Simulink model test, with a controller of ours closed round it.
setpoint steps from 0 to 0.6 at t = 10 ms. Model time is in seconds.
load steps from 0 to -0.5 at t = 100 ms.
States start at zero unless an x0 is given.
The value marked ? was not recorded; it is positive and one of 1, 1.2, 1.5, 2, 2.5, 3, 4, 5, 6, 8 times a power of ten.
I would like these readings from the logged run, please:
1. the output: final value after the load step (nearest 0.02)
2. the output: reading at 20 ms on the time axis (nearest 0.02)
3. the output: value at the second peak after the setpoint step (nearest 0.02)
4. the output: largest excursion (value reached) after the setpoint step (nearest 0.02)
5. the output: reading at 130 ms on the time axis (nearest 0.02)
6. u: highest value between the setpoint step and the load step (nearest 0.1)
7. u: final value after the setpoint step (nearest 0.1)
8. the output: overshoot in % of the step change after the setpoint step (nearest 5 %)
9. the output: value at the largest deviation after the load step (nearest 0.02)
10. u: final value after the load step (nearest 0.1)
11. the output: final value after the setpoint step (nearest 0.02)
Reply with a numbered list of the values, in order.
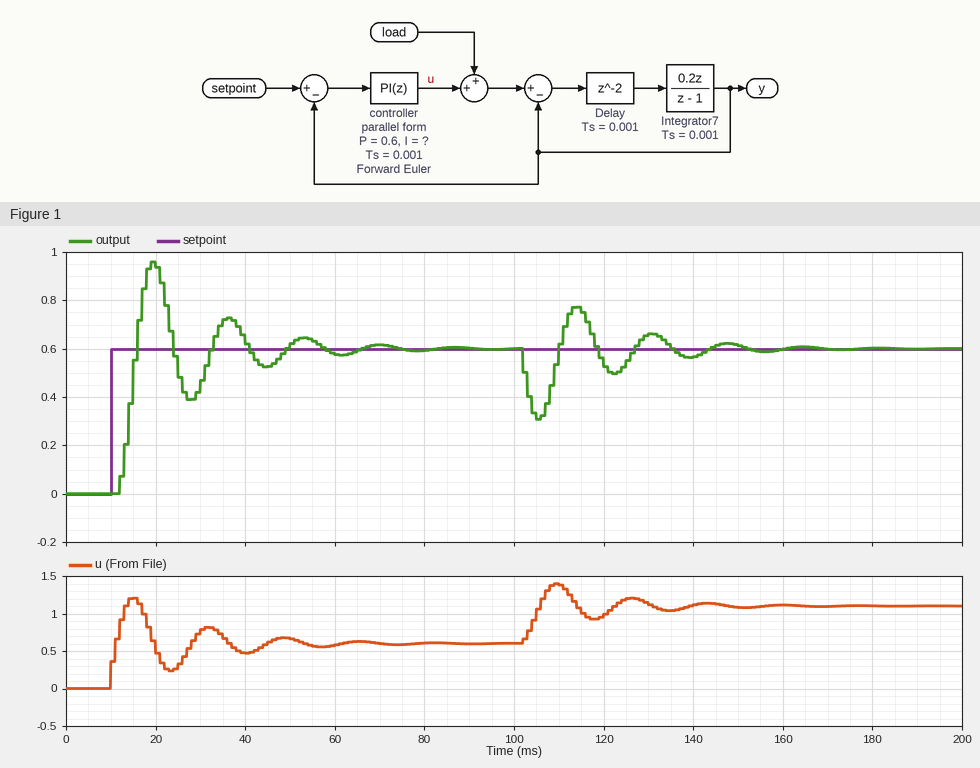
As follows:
1. 0.60
2. 0.94
3. 0.72
4. 0.96
5. 0.66
6. 1.2
7. 0.6
8. 60 %
9. 0.30
10. 1.1
11. 0.60
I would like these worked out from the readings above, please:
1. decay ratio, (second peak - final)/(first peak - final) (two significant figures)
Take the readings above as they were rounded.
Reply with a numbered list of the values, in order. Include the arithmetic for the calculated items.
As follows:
1. (0.72 - 0.6) / (0.96 - 0.6) = 0.33
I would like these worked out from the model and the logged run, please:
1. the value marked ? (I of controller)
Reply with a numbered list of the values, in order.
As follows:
1. 500
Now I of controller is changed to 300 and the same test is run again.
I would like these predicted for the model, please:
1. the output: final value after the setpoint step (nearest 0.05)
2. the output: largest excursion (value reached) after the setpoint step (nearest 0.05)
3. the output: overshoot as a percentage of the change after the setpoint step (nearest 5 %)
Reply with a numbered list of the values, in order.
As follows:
1. 0.60
2. 0.75
3. 20 %
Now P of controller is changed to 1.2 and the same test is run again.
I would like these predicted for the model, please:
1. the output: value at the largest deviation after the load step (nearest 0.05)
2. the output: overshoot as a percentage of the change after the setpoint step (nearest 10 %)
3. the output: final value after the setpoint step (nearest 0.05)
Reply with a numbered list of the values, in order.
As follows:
1. 0.35
2. 40 %
3. 0.60
